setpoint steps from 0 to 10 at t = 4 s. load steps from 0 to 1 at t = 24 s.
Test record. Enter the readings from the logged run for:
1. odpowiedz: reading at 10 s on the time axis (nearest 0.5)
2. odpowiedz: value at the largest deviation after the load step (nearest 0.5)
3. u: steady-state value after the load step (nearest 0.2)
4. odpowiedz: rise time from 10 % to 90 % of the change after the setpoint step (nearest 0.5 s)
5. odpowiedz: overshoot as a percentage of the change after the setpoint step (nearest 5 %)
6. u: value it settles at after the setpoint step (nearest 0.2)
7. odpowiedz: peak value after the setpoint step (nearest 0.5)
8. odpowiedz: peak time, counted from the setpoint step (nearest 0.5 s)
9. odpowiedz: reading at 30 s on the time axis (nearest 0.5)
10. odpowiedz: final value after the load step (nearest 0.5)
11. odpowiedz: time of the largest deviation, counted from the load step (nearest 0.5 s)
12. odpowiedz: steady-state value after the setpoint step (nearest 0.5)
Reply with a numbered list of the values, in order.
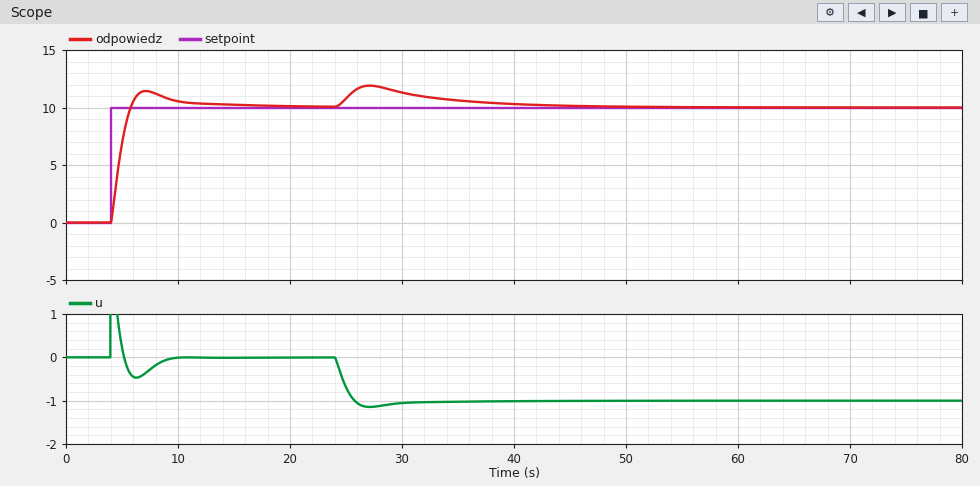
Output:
1. 10.5
2. 12.0
3. -1.0
4. 1.5 s
5. 15 %
6. 0.0
7. 11.5
8. 3.0 s
9. 11.5
10. 10.0
11. 3.0 s
12. 10.0
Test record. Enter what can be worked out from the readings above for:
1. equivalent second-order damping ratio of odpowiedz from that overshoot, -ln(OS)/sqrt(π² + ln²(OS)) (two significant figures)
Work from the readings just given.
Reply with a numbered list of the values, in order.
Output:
1. 0.52
